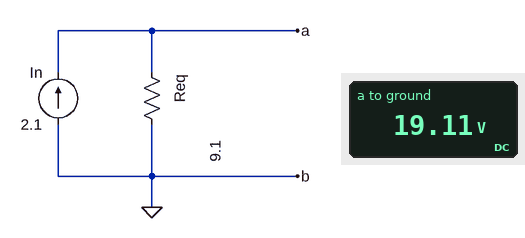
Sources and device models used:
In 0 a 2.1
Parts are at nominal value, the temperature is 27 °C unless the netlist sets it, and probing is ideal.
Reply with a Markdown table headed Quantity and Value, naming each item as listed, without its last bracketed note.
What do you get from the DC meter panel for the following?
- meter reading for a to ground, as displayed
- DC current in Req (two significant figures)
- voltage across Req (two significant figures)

| Quantity | Value |
|---|---|
| meter reading for a to ground, as displayed | 19.11 V |
| DC current in Req | 2.1 A |
| voltage across Req | 19 V |
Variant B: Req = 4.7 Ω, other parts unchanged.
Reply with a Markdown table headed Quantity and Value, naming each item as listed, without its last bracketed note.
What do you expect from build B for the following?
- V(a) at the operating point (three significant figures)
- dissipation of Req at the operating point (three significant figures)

| Quantity | Value |
|---|---|
| V(a) at the operating point | 9.87 V |
| dissipation of Req at the operating point | 20.7 W |
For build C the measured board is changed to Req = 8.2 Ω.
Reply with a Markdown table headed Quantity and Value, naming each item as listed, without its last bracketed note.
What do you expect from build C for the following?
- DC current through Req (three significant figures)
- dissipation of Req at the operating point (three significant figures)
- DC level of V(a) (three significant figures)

| Quantity | Value |
|---|---|
| DC current through Req | 2.10 A |
| dissipation of Req at the operating point | 36.2 W |
| DC level of V(a) | 17.2 V |
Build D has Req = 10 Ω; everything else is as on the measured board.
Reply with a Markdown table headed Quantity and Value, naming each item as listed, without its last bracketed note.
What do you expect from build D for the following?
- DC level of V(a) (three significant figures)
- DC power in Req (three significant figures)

| Quantity | Value |
|---|---|
| DC level of V(a) | 21.0 V |
| DC power in Req | 44.1 W |
